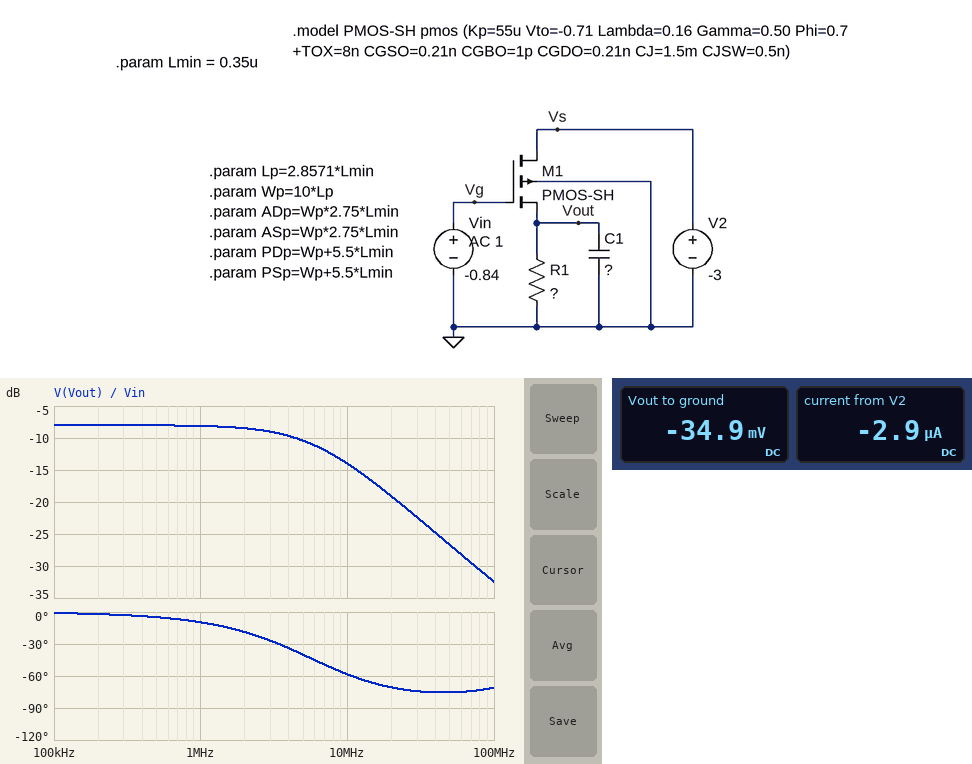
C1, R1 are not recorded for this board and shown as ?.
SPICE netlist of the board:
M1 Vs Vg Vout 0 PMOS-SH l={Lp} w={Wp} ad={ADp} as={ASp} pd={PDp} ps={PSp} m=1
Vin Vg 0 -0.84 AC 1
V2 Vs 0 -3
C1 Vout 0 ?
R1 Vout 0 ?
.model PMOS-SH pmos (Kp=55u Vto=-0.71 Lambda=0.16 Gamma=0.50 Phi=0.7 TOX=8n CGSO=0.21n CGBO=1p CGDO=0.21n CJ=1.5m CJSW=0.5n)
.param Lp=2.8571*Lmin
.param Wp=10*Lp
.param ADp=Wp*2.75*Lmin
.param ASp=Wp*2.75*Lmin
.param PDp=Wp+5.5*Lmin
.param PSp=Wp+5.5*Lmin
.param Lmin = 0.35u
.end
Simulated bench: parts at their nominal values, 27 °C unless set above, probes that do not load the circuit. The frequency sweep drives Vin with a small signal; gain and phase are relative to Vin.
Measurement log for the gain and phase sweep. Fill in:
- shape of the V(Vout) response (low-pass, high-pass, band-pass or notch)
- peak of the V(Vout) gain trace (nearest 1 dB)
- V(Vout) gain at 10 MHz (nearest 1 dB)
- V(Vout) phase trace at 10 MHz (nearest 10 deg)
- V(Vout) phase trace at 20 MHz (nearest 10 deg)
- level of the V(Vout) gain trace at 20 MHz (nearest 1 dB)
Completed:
low-pass
-8 dB
-14 dB
-60 deg
-70 deg
-19 dB
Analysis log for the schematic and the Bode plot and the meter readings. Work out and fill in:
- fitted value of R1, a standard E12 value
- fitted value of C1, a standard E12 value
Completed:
12 kΩ
4.7 pF
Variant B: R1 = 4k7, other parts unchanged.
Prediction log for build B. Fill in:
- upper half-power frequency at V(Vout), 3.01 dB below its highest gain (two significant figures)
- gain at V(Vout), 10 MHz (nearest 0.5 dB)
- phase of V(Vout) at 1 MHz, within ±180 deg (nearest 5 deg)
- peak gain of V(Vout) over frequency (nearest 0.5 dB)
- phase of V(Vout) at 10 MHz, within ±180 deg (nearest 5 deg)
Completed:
11 MHz
-14.5 dB
-5 deg
-11.5 dB
-40 deg
